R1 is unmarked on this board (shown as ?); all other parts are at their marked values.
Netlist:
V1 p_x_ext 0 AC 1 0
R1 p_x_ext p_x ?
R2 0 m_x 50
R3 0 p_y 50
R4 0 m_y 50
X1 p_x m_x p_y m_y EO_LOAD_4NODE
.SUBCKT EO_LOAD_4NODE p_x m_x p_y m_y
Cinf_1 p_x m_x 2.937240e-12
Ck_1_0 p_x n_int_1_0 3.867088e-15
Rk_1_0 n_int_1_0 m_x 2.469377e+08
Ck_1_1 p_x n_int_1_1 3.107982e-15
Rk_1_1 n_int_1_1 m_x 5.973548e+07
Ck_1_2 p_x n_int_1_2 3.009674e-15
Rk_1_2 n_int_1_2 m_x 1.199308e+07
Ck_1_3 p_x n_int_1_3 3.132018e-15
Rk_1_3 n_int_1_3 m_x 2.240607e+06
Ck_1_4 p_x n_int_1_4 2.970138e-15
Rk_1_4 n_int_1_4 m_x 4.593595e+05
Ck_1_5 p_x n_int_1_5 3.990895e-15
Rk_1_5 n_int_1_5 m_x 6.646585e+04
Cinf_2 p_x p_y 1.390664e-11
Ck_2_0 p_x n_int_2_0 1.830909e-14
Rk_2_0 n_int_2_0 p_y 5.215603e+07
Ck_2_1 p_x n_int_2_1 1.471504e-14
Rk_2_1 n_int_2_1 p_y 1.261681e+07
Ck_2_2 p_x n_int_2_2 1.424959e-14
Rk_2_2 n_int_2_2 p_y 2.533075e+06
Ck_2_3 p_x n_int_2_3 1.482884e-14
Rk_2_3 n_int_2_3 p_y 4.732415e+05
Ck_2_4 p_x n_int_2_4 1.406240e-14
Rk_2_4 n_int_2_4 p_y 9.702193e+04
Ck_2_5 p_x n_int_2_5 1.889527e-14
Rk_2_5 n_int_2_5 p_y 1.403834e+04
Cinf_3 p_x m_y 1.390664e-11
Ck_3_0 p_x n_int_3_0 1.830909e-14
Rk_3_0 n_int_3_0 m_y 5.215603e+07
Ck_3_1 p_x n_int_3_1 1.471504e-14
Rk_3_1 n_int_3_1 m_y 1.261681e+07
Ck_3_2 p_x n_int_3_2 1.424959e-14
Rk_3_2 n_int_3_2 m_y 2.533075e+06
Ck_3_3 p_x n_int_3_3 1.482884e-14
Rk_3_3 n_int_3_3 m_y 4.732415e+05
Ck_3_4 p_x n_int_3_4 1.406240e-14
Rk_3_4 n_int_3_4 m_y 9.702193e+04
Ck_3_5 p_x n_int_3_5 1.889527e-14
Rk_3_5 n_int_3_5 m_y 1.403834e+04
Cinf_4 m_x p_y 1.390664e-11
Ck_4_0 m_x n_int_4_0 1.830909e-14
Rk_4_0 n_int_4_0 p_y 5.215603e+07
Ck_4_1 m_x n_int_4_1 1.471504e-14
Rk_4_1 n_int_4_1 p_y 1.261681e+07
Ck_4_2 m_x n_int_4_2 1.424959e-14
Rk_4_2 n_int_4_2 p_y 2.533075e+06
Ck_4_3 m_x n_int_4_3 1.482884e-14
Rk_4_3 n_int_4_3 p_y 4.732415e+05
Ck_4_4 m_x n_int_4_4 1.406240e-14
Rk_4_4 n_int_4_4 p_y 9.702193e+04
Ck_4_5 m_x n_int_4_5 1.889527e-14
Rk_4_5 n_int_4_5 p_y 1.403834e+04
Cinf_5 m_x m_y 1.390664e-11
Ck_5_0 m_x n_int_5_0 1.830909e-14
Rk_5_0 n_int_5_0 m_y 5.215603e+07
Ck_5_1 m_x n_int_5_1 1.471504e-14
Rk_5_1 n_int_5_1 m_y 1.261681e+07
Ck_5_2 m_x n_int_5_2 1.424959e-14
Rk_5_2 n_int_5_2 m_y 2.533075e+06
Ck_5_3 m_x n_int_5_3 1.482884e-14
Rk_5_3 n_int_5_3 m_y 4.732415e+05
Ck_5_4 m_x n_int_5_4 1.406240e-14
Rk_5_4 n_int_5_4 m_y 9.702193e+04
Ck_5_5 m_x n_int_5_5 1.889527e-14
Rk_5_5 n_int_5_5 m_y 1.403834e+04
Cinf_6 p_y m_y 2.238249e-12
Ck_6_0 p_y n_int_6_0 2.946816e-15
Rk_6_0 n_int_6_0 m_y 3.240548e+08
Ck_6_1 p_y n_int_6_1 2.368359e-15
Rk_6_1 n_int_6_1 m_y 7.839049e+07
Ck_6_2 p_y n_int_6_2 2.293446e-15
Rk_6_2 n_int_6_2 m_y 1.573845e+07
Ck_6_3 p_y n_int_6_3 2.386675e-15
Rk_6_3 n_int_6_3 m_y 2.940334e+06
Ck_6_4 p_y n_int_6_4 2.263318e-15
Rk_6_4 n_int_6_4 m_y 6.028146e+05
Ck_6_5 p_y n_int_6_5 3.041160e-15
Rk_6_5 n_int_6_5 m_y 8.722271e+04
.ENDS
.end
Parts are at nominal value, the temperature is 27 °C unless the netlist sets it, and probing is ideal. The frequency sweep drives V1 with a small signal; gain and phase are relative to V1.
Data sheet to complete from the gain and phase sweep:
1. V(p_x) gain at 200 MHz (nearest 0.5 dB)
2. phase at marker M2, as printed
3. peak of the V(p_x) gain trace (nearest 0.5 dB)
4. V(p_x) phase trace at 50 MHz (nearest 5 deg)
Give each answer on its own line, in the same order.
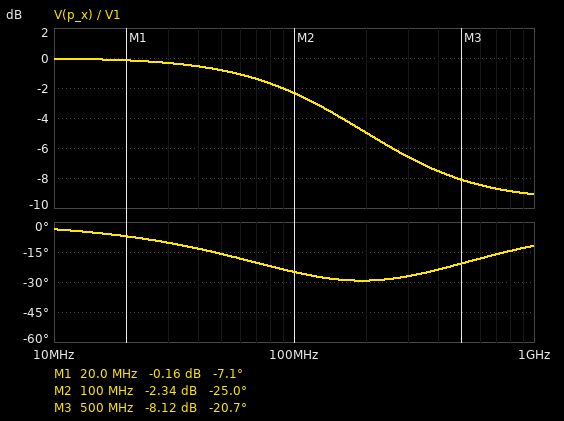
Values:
-5.0 dB
-25.0 deg
0 dB
-15 deg
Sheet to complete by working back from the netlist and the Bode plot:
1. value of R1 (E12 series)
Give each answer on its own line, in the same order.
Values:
33 Ω
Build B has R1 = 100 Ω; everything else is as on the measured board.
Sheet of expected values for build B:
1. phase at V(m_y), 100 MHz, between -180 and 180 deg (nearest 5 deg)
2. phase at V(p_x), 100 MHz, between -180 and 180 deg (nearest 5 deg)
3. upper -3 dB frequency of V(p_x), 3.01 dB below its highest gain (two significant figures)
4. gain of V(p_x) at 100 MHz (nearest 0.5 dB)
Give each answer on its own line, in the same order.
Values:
15 deg
-45 deg
45 MHz
-7.0 dB
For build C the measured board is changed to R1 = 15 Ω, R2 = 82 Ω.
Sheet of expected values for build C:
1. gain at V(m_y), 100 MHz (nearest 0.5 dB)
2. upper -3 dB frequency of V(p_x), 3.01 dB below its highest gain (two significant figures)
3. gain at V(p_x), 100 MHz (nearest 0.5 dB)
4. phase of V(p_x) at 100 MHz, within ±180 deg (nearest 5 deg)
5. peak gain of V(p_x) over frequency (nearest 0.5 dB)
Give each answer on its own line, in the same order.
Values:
-10.0 dB
250 MHz
-1.0 dB
-15 deg
0 dB
